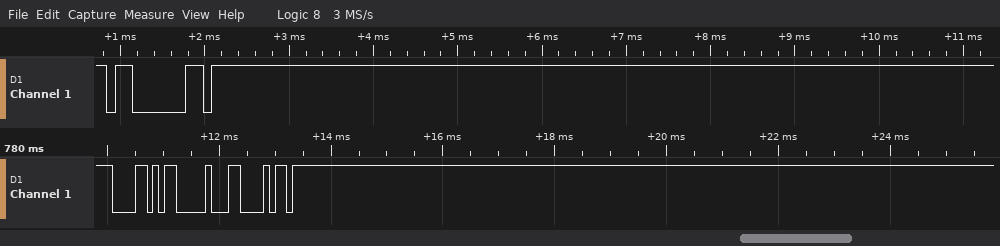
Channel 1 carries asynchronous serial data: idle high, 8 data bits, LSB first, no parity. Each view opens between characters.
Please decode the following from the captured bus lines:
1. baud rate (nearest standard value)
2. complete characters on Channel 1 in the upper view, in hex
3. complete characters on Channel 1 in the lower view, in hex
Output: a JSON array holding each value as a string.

["9600 baud", "03, FF", "58, 10, 68"]
